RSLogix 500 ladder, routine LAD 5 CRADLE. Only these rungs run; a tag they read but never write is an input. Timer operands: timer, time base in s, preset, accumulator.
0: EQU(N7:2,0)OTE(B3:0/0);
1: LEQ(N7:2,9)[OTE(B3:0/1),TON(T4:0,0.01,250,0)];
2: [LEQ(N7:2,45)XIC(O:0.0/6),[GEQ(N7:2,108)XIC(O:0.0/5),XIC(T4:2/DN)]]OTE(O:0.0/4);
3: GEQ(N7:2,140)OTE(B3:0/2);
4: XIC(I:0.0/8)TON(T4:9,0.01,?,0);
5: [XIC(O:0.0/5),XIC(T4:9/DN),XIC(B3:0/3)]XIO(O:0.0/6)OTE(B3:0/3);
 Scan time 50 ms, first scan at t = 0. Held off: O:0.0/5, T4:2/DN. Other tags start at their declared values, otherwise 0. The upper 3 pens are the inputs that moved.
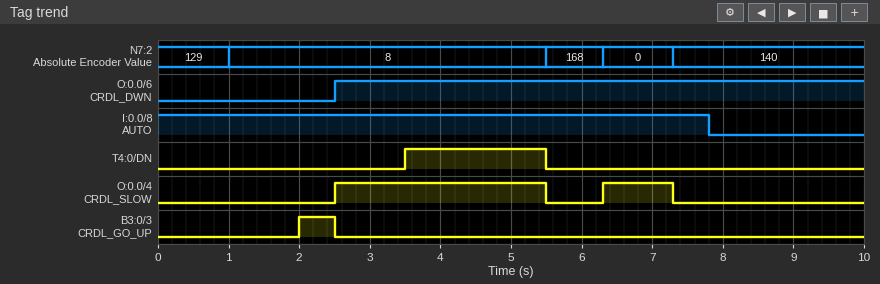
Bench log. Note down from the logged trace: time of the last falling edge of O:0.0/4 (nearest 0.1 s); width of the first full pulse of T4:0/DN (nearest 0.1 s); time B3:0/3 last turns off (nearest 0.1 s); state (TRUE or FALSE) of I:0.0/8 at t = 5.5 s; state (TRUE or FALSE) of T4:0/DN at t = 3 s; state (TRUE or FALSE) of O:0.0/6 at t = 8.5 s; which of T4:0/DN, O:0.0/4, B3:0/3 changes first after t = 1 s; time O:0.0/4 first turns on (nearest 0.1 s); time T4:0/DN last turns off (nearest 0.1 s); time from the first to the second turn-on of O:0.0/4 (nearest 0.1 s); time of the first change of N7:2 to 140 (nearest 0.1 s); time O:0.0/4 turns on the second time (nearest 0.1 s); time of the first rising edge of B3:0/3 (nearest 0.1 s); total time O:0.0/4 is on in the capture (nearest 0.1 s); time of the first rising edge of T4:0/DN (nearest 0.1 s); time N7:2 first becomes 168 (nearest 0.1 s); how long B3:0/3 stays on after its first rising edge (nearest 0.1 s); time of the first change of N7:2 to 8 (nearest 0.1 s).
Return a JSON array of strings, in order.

["7.3 s", "2.0 s", "2.5 s", "TRUE", "FALSE", "TRUE", "B3:0/3", "2.5 s", "5.5 s", "3.8 s", "7.3 s", "6.3 s", "2.0 s", "4.0 s", "3.5 s", "5.5 s", "0.5 s", "1.0 s"]
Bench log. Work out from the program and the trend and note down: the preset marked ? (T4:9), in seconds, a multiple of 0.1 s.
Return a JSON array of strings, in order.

["2.0 s"]
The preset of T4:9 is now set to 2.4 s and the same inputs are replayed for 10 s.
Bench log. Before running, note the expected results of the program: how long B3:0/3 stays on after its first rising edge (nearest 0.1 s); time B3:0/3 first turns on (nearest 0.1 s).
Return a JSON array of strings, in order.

["0.1 s", "2.4 s"]
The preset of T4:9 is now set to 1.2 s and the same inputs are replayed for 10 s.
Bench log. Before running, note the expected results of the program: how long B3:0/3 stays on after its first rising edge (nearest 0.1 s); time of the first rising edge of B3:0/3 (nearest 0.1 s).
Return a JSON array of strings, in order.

["1.3 s", "1.2 s"]
